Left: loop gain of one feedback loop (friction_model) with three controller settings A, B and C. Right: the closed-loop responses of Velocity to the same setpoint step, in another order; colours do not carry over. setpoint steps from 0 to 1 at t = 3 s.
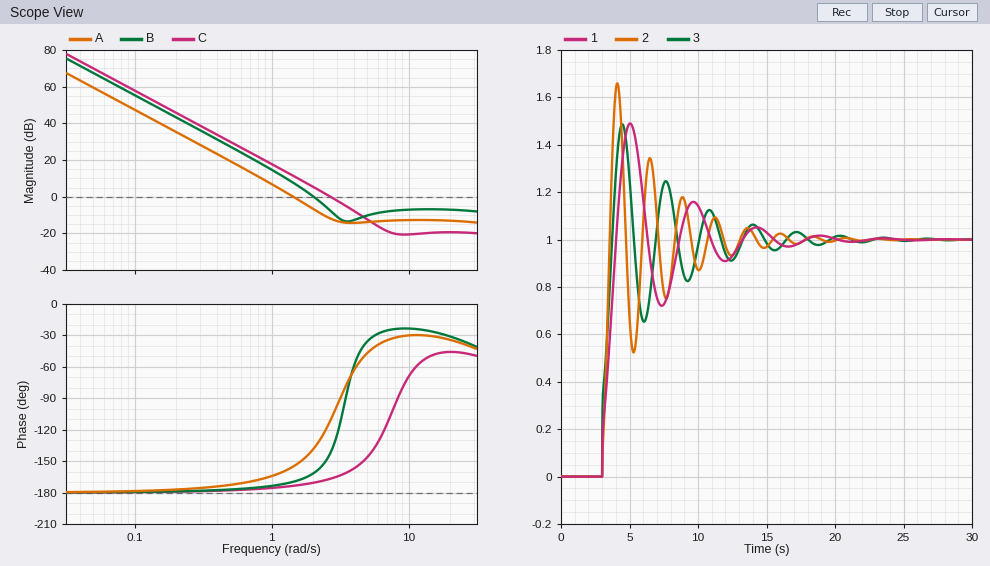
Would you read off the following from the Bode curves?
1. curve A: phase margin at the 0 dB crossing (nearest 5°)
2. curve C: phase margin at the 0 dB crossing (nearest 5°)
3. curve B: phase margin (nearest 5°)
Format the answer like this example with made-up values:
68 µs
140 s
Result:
25°
15°
20°
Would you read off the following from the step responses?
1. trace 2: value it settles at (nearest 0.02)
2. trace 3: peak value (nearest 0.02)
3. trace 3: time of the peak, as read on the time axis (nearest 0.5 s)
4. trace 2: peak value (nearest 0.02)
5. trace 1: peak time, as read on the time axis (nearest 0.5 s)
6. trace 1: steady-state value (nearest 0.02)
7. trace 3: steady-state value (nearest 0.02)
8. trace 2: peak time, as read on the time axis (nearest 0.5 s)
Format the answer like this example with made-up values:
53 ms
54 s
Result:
1.00
1.48
4.5 s
1.66
5.0 s
1.00
1.00
4.0 s
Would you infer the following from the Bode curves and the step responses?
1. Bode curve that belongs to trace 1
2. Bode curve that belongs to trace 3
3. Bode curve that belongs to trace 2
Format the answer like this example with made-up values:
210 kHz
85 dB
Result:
A
B
C
